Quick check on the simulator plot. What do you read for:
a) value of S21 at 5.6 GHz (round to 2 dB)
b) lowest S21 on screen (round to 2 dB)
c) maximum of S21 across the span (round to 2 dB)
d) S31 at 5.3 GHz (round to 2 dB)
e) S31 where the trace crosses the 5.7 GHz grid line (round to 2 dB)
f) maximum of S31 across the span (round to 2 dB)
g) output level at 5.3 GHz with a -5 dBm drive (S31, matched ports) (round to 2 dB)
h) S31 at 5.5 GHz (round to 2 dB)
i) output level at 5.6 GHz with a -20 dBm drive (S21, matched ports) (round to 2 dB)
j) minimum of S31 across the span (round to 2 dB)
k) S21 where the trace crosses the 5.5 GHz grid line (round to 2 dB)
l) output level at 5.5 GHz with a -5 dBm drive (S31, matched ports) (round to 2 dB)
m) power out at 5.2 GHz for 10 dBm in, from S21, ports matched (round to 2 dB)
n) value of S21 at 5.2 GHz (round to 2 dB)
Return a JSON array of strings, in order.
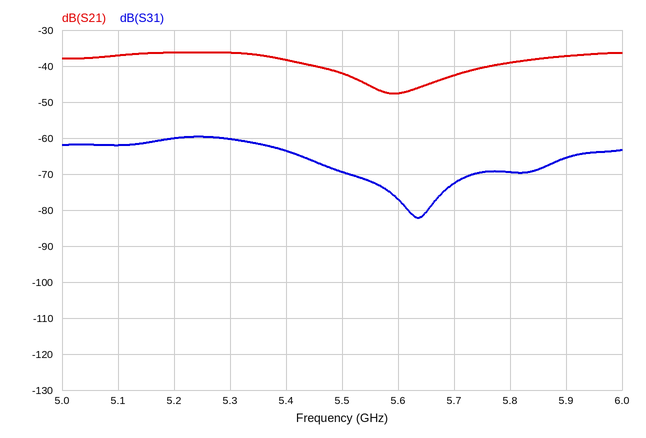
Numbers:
["-48 dB", "-48 dB", "-36 dB", "-60 dB", "-72 dB", "-60 dB", "-66 dBm", "-70 dB", "-68 dBm", "-82 dB", "-42 dB", "-74 dBm", "-26 dBm", "-36 dB"]
